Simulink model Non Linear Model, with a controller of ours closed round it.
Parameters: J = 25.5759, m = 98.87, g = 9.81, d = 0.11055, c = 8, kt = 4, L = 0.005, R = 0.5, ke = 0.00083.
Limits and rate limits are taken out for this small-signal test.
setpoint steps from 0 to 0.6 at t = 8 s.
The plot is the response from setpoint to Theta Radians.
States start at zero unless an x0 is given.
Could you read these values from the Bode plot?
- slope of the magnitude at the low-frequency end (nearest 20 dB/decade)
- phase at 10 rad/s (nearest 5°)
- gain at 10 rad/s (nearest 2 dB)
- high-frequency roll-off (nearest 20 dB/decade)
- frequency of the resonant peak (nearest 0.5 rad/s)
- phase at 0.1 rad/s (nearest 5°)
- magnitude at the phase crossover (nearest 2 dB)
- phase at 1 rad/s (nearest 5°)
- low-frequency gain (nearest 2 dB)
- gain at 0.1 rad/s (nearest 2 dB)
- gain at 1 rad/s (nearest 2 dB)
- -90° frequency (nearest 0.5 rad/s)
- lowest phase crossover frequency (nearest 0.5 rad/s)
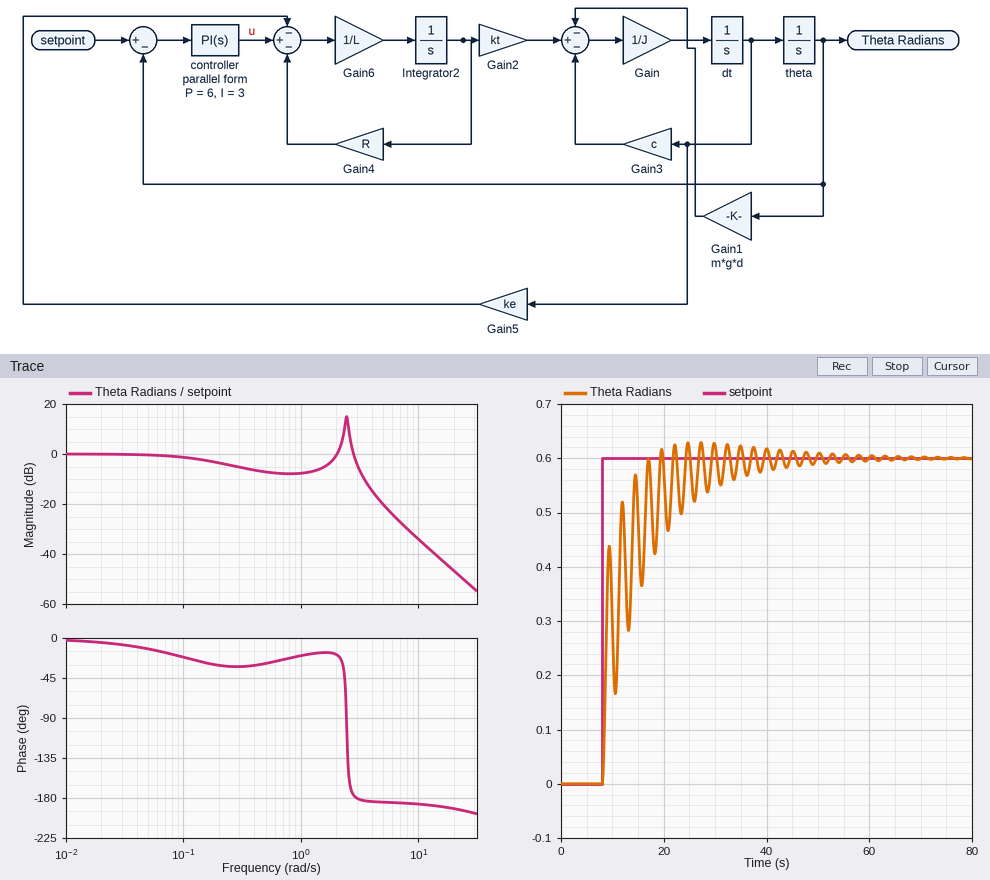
0 dB/decade
-185°
-34 dB
-40 dB/decade
2.5 rad/s
-20°
-4 dB
-20°
0 dB
-2 dB
-8 dB
2.5 rad/s
3.0 rad/s
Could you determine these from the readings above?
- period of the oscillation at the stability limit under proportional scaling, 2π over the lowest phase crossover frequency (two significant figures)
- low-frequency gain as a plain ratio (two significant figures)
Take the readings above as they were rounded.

2.1 s
1.0
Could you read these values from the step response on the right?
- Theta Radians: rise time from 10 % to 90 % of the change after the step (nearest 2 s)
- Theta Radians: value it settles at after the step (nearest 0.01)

6 s
0.60
